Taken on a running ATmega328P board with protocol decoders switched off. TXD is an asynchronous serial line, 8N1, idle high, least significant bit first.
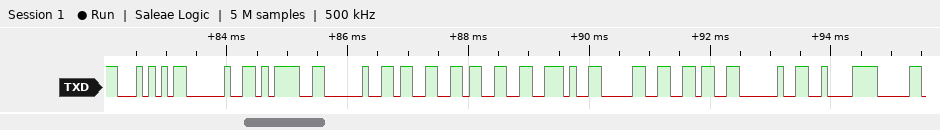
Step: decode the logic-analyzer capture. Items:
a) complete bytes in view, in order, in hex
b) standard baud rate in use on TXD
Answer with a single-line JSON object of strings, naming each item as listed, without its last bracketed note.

{"complete bytes in view, in order, in hex": "0x54 0x20 0x3D 0x20 0x33 0x33 0x2E 0x30 0x36 0x20 0xC2", "standard baud rate in use on TXD": "9600 baud"}
